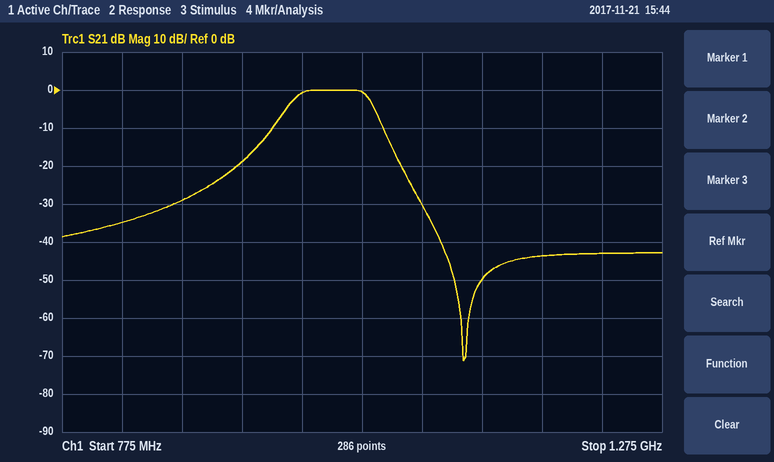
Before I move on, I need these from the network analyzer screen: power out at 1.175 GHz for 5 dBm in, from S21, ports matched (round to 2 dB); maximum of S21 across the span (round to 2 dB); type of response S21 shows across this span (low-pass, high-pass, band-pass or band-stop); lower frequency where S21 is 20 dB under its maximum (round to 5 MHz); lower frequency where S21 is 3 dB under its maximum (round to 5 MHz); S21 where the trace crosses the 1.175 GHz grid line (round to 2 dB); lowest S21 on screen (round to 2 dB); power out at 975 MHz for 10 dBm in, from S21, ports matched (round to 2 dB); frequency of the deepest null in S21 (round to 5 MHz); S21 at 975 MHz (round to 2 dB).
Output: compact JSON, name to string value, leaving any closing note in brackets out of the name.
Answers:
{"power out at 1.175 GHz for 5 dBm in, from S21, ports matched": "-38 dBm", "maximum of S21 across the span": "0 dB", "type of response S21 shows across this span": "band-pass", "lower frequency where S21 is 20 dB under its maximum": "920 MHz", "lower frequency where S21 is 3 dB under its maximum": "965 MHz", "S21 where the trace crosses the 1.175 GHz grid line": "-44 dB", "lowest S21 on screen": "-72 dB", "power out at 975 MHz for 10 dBm in, from S21, ports matched": "10 dBm", "frequency of the deepest null in S21": "1.110 GHz", "S21 at 975 MHz": "0 dB"}
